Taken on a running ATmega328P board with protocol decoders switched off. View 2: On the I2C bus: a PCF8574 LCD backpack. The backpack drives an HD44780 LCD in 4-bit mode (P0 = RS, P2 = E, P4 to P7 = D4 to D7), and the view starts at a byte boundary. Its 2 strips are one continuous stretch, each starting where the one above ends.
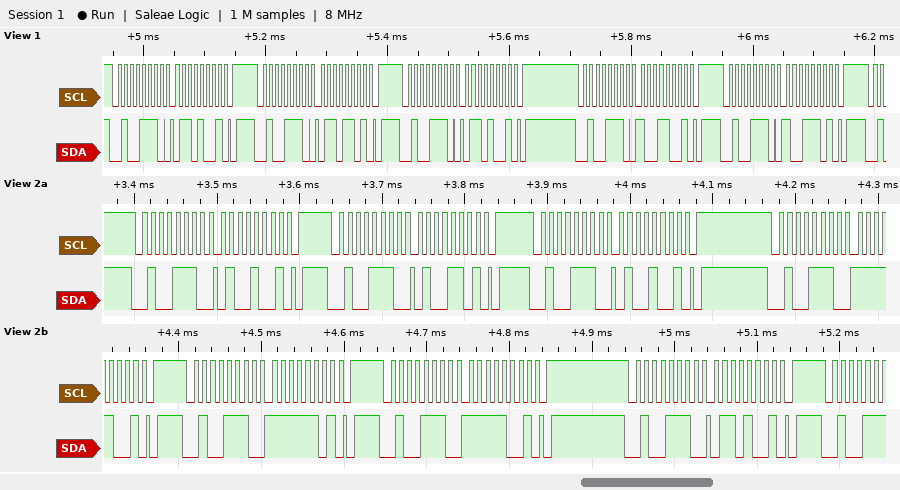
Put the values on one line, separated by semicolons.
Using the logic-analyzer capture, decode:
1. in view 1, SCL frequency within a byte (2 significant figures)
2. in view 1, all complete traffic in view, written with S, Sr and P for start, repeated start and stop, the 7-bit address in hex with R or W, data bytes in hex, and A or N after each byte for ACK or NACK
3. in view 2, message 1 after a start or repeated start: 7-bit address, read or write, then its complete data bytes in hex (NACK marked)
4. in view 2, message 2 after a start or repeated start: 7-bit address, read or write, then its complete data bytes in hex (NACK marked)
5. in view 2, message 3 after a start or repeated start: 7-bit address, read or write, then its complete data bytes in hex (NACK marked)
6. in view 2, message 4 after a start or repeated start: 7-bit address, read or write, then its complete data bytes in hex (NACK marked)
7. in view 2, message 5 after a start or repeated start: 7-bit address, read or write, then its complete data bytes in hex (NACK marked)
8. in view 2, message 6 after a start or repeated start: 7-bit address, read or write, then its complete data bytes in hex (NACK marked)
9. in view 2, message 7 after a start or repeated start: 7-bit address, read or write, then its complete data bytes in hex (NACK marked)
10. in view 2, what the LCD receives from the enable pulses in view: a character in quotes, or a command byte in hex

100 kHz; S 27W A 69 A P S 27W A 6D A P S 27W A 69 A P S 27W A 99 A P S 27W A 9D A P; 0x27 write: 49; 0x27 write: 4D; 0x27 write: 49; 0x27 write: F9; 0x27 write: FD; 0x27 write: F9; 0x27 write: 69; 'O'
